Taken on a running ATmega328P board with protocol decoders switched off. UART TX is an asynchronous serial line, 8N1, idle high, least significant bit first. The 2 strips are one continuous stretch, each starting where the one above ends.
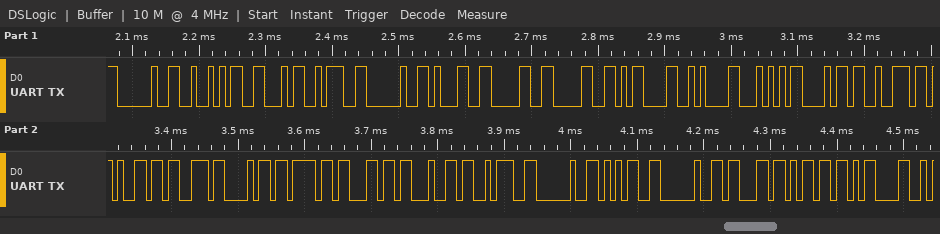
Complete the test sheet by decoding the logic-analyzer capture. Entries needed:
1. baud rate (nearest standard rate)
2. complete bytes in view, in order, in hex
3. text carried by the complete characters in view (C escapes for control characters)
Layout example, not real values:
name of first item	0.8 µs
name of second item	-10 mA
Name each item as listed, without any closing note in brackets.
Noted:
baud rate	115200 baud
complete bytes in view, in order, in hex	20 52 46 3A 20 31 30 30 0D 0A 54 68 72 65 73 68 6F 6C 64 3A 20 35 20 63 6D 0D
text carried by the complete characters in view	" RF: 100\r\nThreshold: 5 cm\r"
